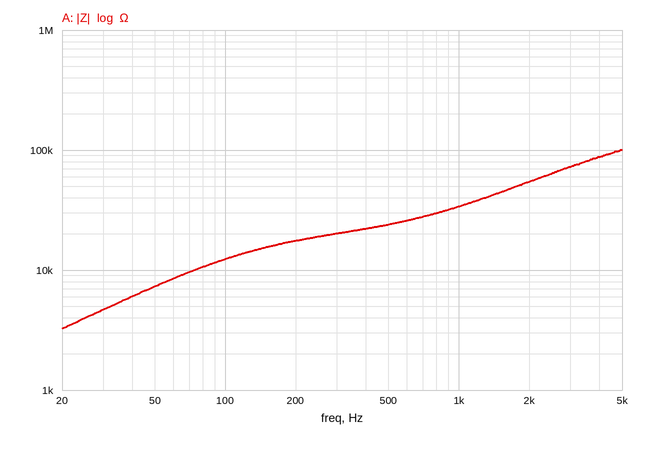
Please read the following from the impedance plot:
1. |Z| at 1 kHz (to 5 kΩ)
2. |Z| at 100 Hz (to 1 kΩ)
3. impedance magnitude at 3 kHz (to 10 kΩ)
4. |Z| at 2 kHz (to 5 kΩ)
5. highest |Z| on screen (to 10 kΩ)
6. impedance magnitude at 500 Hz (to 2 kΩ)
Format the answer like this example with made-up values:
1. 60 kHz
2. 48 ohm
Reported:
1. 35 kΩ
2. 12 kΩ
3. 70 kΩ
4. 55 kΩ
5. 100 kΩ
6. 24 kΩ
